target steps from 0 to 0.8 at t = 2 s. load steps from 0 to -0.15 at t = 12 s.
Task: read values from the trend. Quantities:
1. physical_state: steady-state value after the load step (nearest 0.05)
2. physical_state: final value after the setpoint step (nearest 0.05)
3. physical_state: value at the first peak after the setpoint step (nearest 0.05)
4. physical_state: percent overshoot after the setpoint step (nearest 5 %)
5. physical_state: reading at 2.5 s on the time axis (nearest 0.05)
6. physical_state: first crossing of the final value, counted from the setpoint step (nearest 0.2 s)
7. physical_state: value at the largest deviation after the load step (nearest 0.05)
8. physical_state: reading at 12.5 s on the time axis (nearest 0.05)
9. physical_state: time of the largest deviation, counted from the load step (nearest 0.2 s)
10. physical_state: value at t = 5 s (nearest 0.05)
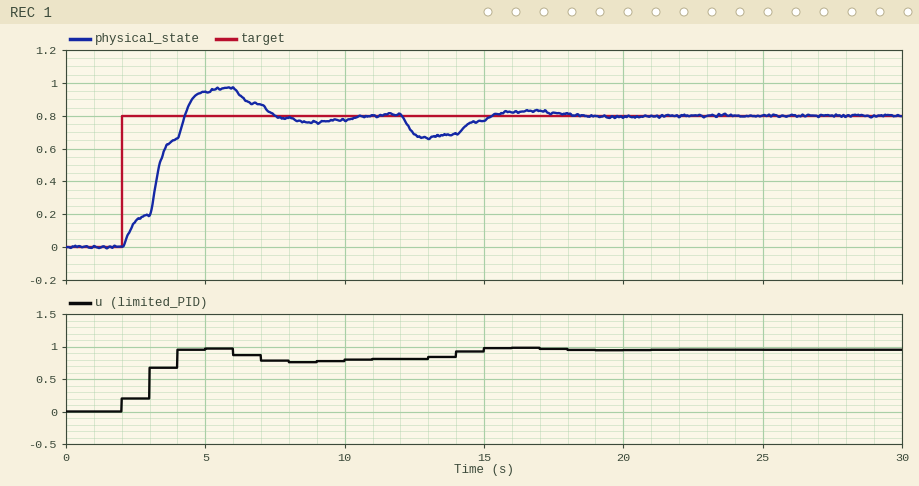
0.80
0.80
0.95
20 %
0.15
2.2 s
0.65
0.70
1.0 s
0.95
